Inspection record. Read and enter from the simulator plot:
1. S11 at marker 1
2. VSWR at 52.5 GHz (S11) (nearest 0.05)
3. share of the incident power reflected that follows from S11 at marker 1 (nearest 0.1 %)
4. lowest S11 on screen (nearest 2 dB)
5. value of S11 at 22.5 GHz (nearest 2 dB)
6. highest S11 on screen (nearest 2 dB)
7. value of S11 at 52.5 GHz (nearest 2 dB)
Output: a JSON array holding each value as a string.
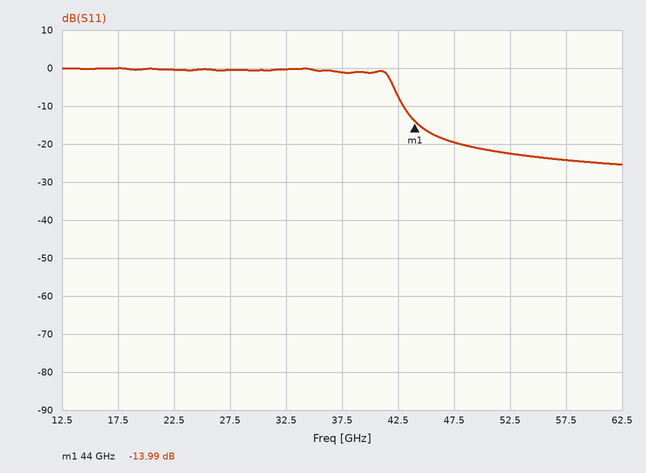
["-13.99 dB", "1.15", "4.0 %", "-26 dB", "0 dB", "0 dB", "-22 dB"]
